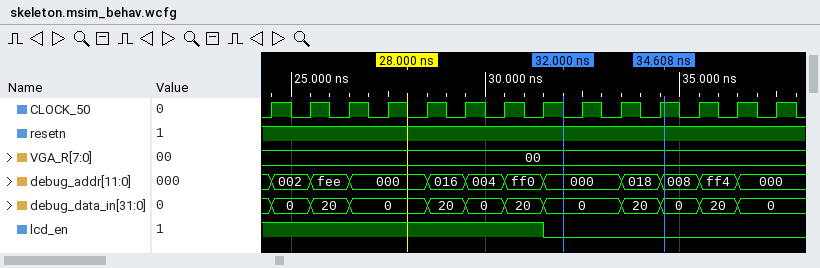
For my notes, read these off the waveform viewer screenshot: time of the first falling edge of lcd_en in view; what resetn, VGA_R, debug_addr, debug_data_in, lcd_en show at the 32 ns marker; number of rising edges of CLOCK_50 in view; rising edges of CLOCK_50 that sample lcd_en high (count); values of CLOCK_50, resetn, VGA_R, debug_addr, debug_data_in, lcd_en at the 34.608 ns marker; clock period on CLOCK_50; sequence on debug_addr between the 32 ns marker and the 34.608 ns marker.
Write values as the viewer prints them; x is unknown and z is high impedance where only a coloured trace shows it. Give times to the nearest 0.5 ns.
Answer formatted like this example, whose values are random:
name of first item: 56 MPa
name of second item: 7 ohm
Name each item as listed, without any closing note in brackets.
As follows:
time of the first falling edge of lcd_en in view: 31.5 ns
what resetn, VGA_R, debug_addr, debug_data_in, lcd_en show at the 32 ns marker: resetn=1, VGA_R=00, debug_addr=000, debug_data_in=0, lcd_en=0
number of rising edges of CLOCK_50 in view: 14
rising edges of CLOCK_50 that sample lcd_en high: 8
values of CLOCK_50, resetn, VGA_R, debug_addr, debug_data_in, lcd_en at the 34.608 ns marker: CLOCK_50=1, resetn=1, VGA_R=00, debug_addr=008, debug_data_in=0, lcd_en=0
clock period on CLOCK_50: 1 ns
sequence on debug_addr between the 32 ns marker and the 34.608 ns marker: 000, 018, 008
